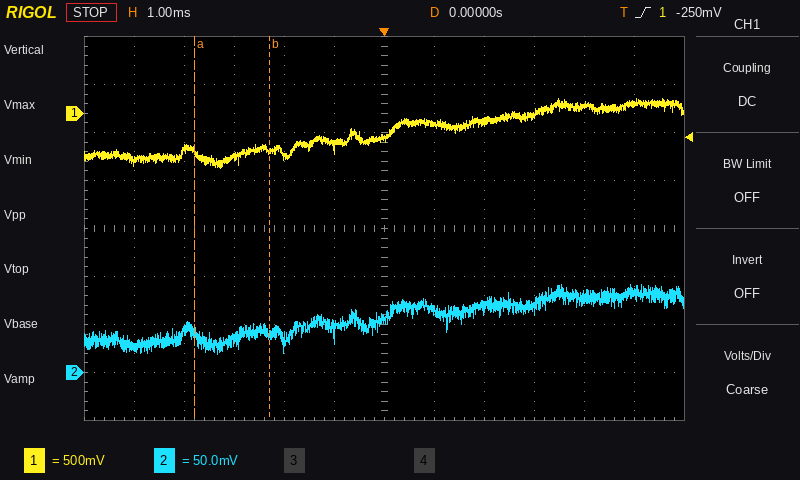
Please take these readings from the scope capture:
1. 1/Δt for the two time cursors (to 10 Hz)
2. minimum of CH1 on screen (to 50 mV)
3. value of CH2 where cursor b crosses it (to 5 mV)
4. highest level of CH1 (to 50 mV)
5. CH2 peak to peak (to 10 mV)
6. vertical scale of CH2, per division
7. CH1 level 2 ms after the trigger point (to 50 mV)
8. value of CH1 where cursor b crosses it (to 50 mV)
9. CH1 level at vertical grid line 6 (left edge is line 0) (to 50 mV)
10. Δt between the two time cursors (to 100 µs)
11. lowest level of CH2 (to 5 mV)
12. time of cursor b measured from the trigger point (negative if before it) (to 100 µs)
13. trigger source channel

670 Hz
-550 mV
40 mV
150 mV
70 mV
50 mV
-100 mV
-400 mV
-250 mV
1.5 ms
20 mV
-2.3 ms
CH1
